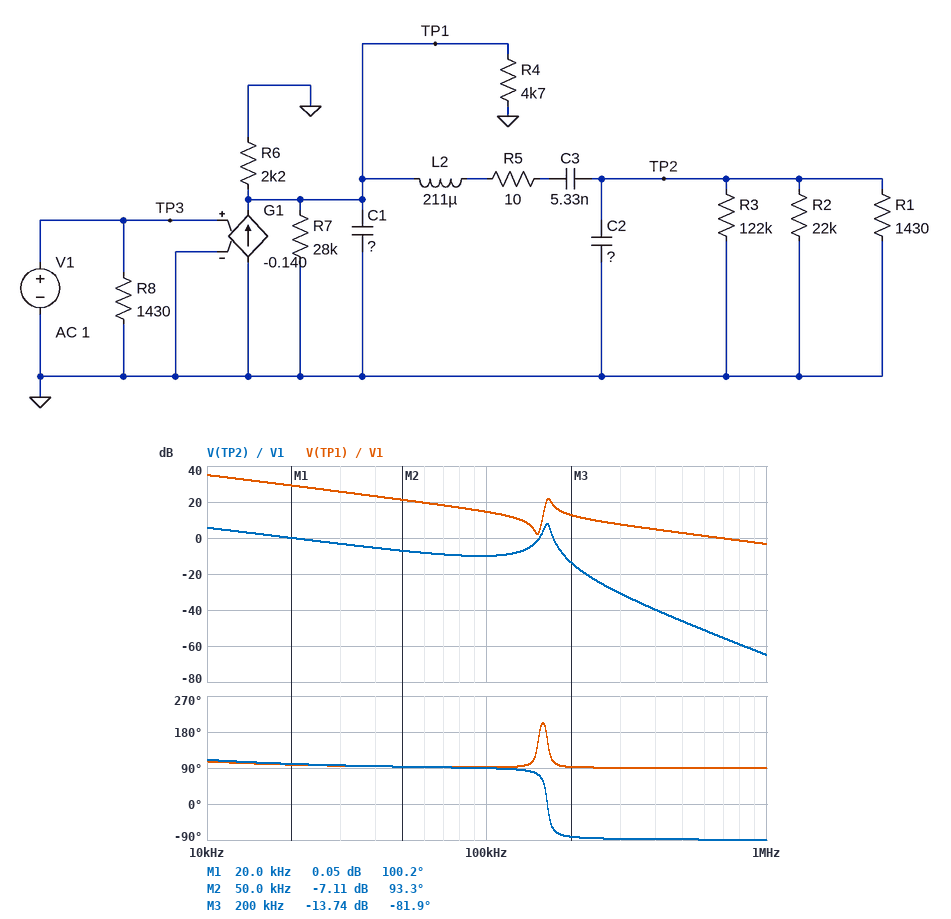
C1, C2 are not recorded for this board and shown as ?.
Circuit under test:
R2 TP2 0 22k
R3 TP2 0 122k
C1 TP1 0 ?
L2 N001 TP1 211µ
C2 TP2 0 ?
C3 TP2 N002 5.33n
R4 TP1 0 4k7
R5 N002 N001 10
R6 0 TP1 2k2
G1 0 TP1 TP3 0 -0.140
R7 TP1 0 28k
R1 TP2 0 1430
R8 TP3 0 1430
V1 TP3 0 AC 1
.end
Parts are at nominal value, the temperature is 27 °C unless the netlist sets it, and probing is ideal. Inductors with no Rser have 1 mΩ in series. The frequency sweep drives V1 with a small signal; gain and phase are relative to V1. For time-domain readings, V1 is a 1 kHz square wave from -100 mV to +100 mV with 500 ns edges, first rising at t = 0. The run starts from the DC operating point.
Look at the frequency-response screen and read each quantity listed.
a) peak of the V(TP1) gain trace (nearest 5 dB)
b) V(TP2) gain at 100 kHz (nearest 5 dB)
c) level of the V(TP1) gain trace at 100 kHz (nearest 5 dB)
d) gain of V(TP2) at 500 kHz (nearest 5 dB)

35 dB
-10 dB
15 dB
-45 dB
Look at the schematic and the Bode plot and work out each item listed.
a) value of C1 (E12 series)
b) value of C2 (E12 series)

33 nF
150 nF
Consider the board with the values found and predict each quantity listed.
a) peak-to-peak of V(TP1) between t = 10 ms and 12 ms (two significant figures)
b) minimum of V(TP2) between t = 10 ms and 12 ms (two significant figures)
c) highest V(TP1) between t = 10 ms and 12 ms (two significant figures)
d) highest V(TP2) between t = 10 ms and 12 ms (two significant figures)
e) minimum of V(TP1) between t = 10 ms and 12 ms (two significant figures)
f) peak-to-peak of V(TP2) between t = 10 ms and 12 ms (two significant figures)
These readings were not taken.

40 V
-760 mV
20 V
760 mV
-20 V
1.5 V
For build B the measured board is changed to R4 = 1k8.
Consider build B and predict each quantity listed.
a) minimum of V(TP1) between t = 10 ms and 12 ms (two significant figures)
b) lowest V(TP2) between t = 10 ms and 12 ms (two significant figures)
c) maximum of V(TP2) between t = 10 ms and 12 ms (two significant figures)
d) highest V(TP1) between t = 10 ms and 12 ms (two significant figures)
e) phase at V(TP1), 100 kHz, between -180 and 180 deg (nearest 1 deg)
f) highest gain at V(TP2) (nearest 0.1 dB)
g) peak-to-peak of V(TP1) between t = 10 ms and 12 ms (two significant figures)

-13 V
-570 mV
570 mV
13 V
93 deg
11.8 dB
27 V
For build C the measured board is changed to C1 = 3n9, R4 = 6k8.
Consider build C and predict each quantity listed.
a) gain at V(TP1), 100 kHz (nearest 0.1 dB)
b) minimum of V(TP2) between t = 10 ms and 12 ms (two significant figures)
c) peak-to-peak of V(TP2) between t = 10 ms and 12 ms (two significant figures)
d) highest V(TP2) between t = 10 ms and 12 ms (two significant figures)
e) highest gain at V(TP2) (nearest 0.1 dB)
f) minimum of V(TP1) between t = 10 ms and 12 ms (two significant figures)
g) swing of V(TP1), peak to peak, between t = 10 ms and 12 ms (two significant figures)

24.7 dB
-1.1 V
2.3 V
1.1 V
17.0 dB
-22 V
44 V
